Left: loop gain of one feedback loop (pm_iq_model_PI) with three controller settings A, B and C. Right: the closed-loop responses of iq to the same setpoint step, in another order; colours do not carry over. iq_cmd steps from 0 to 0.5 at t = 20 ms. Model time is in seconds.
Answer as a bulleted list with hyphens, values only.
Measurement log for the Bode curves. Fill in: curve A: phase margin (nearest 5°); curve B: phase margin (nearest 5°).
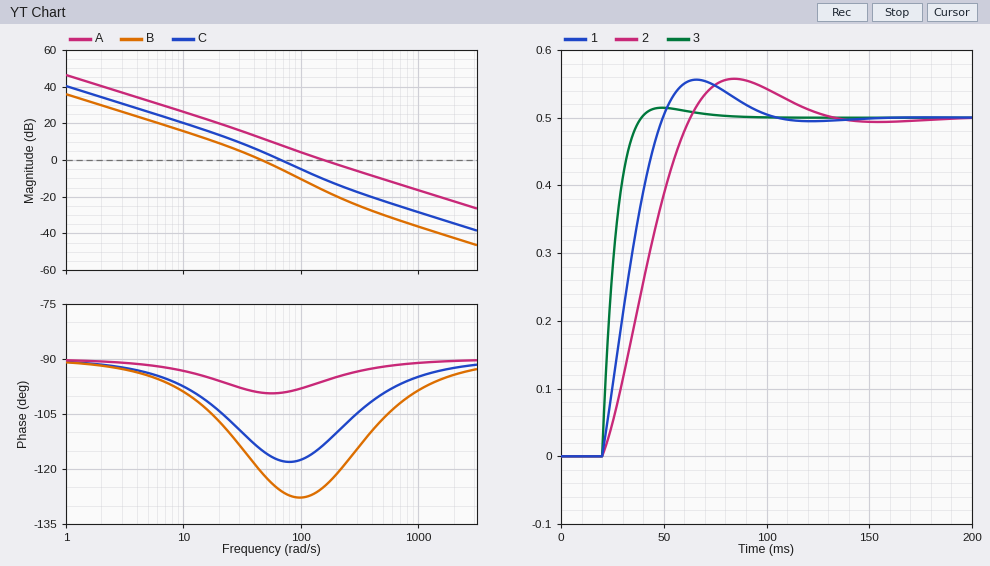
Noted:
- 85°
- 60°
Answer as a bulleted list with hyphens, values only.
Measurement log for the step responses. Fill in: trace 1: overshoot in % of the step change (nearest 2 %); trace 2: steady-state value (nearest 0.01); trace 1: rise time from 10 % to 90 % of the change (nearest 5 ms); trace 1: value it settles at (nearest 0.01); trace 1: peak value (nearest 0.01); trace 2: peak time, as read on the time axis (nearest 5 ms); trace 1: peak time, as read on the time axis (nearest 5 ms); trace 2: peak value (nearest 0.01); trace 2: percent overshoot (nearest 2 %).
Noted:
- 12 %
- 0.50
- 20 ms
- 0.50
- 0.56
- 85 ms
- 65 ms
- 0.56
- 12 %
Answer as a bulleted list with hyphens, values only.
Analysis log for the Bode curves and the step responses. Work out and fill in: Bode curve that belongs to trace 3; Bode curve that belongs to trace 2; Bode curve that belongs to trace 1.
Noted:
- A
- B
- C
